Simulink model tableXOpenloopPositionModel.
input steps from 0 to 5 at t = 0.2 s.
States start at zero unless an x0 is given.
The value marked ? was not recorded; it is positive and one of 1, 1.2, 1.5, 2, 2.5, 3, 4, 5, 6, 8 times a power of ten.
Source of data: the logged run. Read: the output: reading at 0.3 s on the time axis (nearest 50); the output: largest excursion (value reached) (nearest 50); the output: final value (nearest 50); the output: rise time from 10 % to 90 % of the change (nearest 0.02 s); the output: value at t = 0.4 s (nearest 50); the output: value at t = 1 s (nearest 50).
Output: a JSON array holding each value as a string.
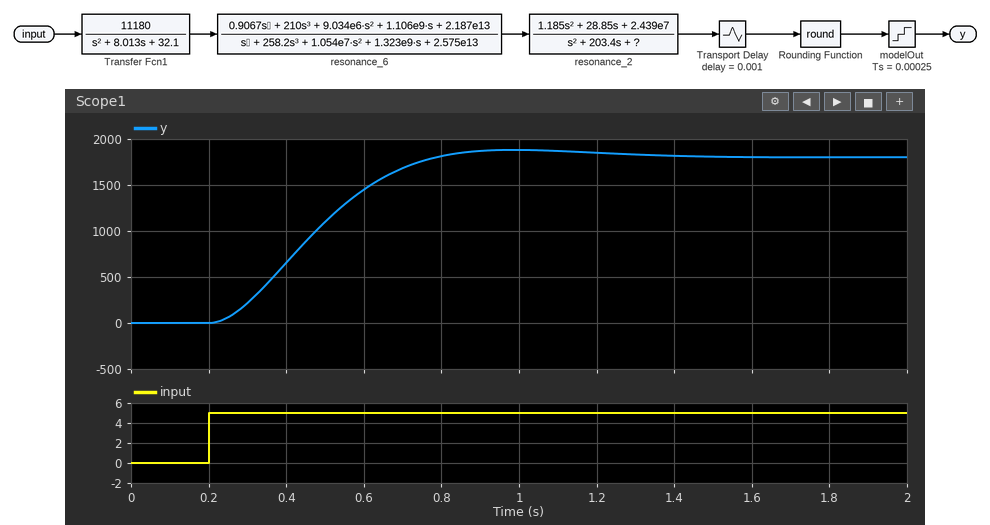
["200", "1900", "1800", "0.38 s", "650", "1900"]
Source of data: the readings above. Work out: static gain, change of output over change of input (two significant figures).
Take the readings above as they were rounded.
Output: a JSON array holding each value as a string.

["360"]
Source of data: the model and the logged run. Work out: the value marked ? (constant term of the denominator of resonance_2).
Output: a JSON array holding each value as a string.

["2e+07"]
